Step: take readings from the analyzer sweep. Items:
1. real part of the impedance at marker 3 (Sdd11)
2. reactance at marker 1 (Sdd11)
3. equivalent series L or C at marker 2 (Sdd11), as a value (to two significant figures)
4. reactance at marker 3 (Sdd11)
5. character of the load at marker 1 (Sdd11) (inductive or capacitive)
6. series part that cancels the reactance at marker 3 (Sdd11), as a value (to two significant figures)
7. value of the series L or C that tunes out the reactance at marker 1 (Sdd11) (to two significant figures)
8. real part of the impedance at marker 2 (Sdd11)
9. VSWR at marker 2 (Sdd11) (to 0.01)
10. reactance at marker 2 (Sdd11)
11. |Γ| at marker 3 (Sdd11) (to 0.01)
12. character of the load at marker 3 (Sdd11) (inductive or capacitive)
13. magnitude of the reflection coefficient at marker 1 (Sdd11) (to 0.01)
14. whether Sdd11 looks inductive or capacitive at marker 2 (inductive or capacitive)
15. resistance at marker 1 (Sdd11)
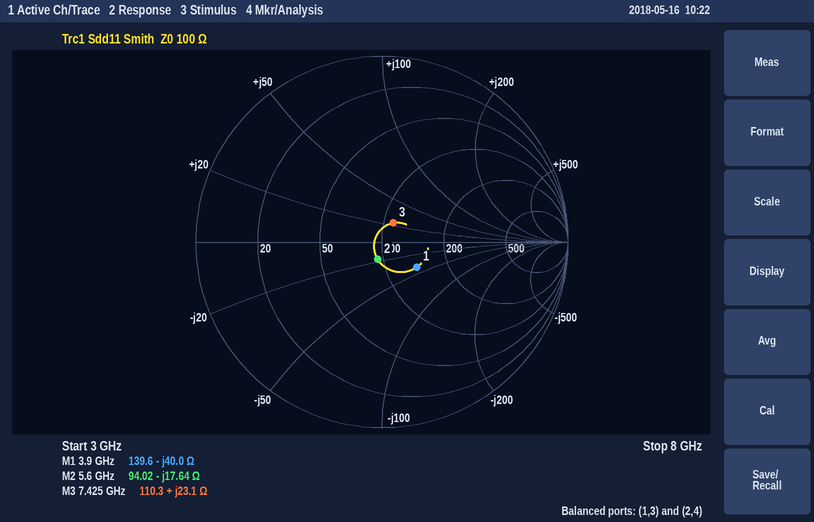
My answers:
110.3 Ω
-40.0 Ω
1.6 pF
+23.1 Ω
capacitive
930 fF
1.6 nH
94.02 Ω
1.21
-17.64 Ω
0.12
inductive
0.23
capacitive
139.6 Ω
